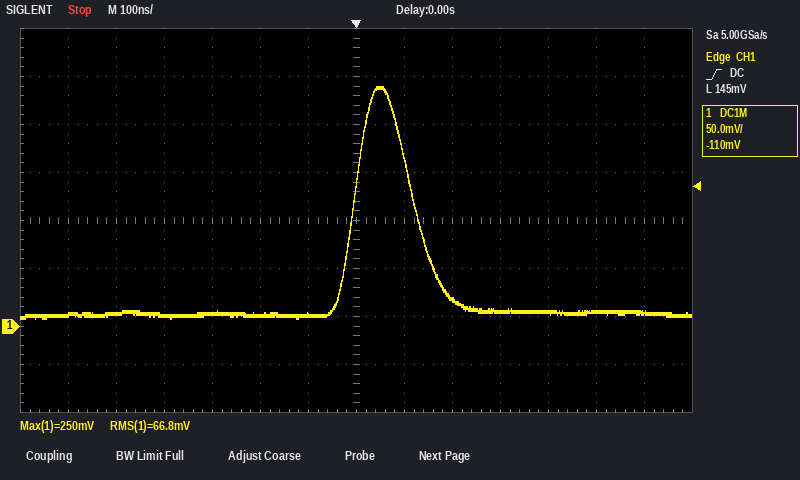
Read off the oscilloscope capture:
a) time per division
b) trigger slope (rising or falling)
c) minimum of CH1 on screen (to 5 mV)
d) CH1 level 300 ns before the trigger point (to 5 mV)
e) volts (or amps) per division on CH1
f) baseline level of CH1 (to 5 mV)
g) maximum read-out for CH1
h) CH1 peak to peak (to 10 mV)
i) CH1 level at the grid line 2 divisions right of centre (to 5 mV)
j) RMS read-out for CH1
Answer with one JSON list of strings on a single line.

["100 ns", "rising", "10 mV", "15 mV", "50 mV", "15 mV", "250 mV", "240 mV", "30 mV", "66.8 mV"]
